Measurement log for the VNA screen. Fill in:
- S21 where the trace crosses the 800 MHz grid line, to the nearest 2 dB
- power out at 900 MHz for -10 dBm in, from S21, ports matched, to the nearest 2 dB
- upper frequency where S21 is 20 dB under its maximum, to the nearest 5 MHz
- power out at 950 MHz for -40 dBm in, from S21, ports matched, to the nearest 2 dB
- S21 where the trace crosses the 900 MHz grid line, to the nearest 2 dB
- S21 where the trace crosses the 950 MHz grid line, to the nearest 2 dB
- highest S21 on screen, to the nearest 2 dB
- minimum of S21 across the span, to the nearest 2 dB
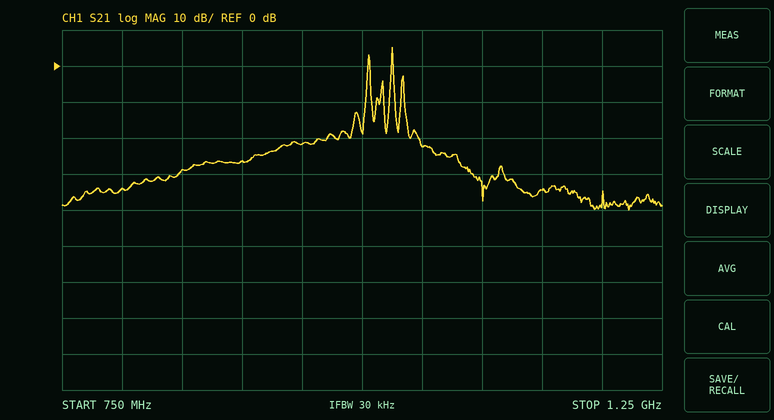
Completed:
-34 dB
-36 dBm
1.030 GHz
-62 dBm
-26 dB
-22 dB
6 dB
-40 dB
